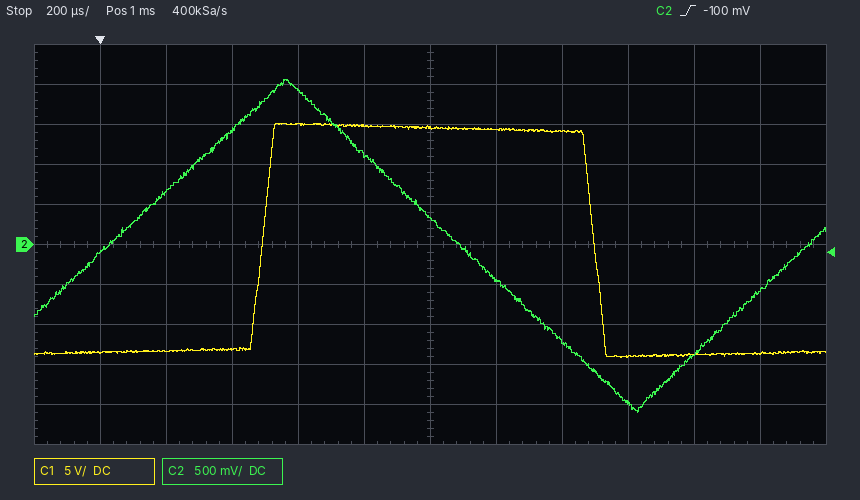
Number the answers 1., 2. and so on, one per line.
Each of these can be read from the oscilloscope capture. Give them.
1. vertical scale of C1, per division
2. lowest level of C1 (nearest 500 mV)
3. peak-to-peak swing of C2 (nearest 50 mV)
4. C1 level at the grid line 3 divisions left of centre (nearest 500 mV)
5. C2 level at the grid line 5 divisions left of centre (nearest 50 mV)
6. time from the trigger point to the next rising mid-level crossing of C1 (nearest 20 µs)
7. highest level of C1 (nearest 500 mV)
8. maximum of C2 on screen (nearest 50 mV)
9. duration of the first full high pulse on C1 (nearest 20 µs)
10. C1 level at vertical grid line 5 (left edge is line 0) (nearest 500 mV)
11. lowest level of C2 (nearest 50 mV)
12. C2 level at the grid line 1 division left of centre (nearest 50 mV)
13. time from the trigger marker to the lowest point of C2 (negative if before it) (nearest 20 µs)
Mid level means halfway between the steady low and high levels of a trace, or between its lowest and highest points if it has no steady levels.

1. 5 V
2. -14.0 V
3. 4.15 V
4. -13.0 V
5. -100 mV
6. 500 µs
7. 15.0 V
8. 2.05 V
9. 1.00 ms
10. 15.0 V
11. -2.10 V
12. 1.15 V
13. +1.62 ms
